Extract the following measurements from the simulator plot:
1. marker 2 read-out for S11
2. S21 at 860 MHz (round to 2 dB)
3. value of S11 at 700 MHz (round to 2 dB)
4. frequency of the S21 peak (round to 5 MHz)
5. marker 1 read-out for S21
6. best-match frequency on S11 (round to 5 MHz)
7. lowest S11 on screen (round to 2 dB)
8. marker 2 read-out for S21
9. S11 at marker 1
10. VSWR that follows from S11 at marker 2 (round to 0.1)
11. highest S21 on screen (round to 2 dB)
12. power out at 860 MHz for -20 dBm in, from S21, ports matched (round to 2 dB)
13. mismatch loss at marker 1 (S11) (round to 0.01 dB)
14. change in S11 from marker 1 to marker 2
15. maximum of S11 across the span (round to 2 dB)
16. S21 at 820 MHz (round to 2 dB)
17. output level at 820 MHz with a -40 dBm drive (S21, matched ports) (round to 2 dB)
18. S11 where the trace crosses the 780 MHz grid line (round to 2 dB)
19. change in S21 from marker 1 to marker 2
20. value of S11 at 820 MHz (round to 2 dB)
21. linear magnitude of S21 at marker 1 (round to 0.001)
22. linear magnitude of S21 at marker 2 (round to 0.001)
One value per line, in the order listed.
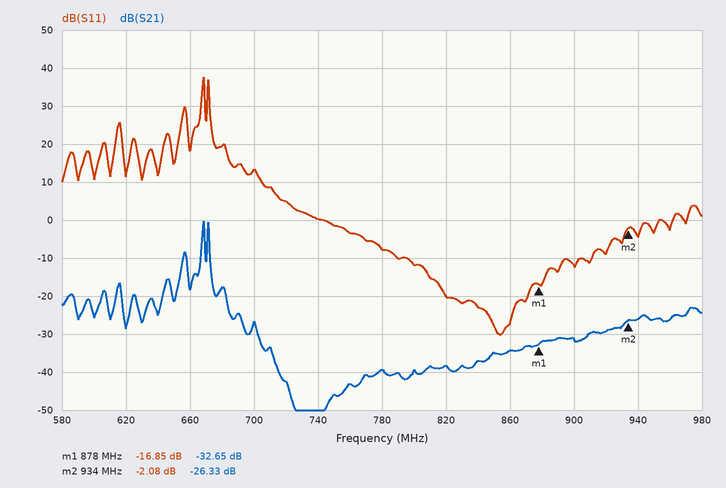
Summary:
-2.08 dB
-34 dB
14 dB
670 MHz
-32.65 dB
855 MHz
-30 dB
-26.33 dB
-16.85 dB
8.4
0 dB
-54 dBm
0.09 dB
14.77 dB
38 dB
-38 dB
-78 dBm
-8 dB
6.32 dB
-20 dB
0.023
0.048
